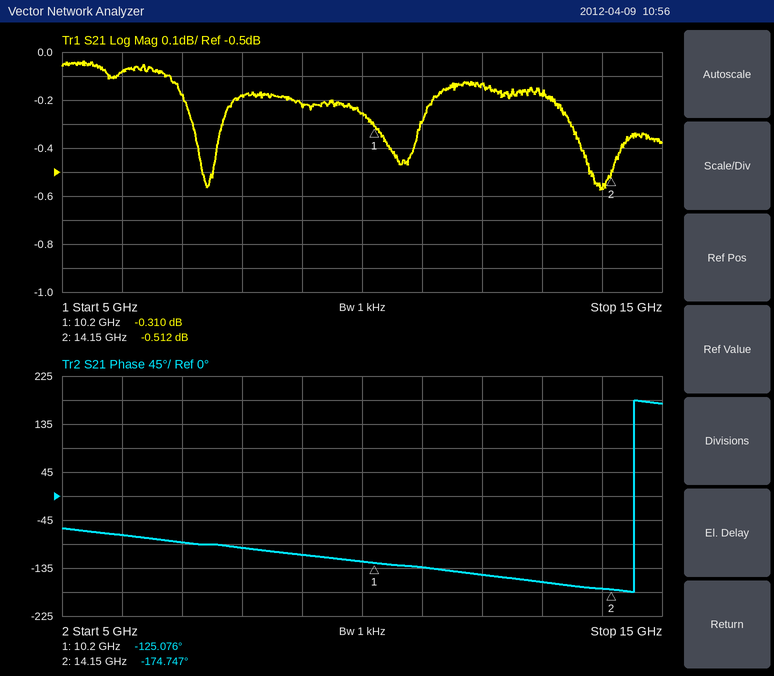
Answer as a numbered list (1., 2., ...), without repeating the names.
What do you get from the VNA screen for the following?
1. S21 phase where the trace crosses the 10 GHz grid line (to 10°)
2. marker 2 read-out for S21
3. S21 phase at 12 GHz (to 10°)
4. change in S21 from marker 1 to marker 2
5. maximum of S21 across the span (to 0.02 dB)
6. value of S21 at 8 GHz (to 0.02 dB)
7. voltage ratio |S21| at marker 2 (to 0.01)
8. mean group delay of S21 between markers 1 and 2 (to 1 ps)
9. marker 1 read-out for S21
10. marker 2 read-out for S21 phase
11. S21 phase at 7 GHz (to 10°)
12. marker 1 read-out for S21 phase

1. -120°
2. -0.512 dB
3. -150°
4. -0.202 dB
5. -0.04 dB
6. -0.18 dB
7. 0.94
8. 35 ps
9. -0.310 dB
10. -174.747°
11. -90°
12. -125.076°
